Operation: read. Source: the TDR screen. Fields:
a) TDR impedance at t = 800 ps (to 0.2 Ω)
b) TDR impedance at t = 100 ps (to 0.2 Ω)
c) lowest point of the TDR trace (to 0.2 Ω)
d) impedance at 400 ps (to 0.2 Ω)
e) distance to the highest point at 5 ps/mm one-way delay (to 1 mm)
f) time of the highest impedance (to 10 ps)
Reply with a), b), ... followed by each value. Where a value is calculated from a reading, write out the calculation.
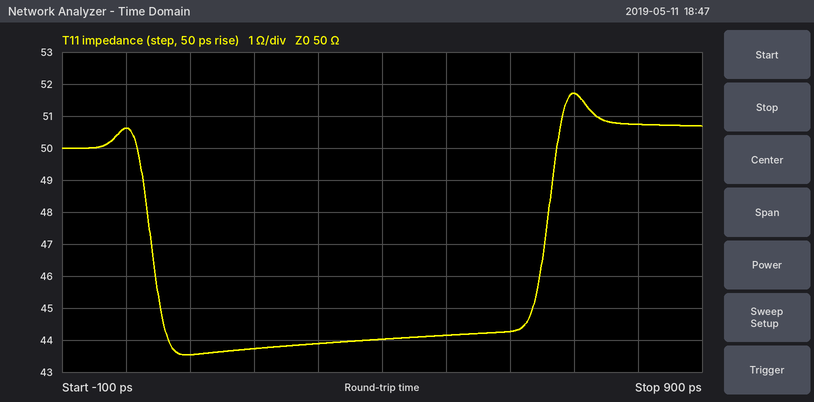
a) 50.8 Ω
b) 43.6 Ω
c) 43.6 Ω
d) 44.0 Ω
e) 700 ps / 2 / 5 ps/mm ≈ 70 mm
f) 700 ps
